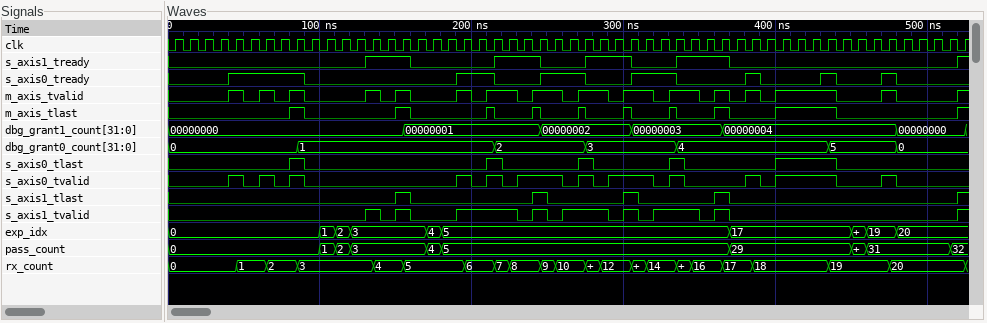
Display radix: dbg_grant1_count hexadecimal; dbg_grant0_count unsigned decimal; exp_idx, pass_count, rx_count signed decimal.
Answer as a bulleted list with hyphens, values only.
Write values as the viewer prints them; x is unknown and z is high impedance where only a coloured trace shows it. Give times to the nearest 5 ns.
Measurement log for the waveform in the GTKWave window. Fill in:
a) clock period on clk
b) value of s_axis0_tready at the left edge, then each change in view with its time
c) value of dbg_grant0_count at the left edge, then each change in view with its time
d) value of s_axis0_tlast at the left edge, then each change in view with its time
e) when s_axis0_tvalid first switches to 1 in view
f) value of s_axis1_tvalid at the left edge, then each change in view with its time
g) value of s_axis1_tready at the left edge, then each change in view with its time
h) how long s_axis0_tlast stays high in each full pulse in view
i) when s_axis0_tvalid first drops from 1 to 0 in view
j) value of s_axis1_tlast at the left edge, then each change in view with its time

- 10 ns
- 0, 1 at 40 ns, 0 at 90 ns, 1 at 190 ns, 0 at 215 ns, 1 at 245 ns, 0 at 275 ns, 1 at 305 ns, 0 at 335 ns, 1 at 380 ns, 0 at 390 ns, 1 at 430 ns, 0 at 440 ns, 1 at 470 ns, 0 at 480 ns
- 0, 1 at 85 ns, 2 at 215 ns, 3 at 275 ns, 4 at 335 ns, 5 at 435 ns, 0 at 480 ns
- 0, 1 at 80 ns, 0 at 90 ns, 1 at 210 ns, 0 at 220 ns, 1 at 270 ns, 0 at 280 ns, 1 at 330 ns, 0 at 340 ns, 1 at 400 ns, 0 at 440 ns
- 40 ns
- 0, 1 at 130 ns, 0 at 140 ns, 1 at 150 ns, 0 at 160 ns, 1 at 190 ns, 0 at 230 ns, 1 at 240 ns, 0 at 250 ns, 1 at 260 ns, 0 at 290 ns, 1 at 300 ns, 0 at 310 ns, 1 at 320 ns, 0 at 350 ns, 1 at 360 ns, 0 at 370 ns, 1 at 520 ns
- 0, 1 at 130 ns, 0 at 160 ns, 1 at 215 ns, 0 at 245 ns, 1 at 275 ns, 0 at 305 ns, 1 at 335 ns, 0 at 370 ns, 1 at 520 ns
- 10 ns, 10 ns, 10 ns, 10 ns, 40 ns
- 50 ns
- 0, 1 at 150 ns, 0 at 160 ns, 1 at 240 ns, 0 at 250 ns, 1 at 300 ns, 0 at 310 ns, 1 at 360 ns, 0 at 370 ns, 1 at 520 ns
